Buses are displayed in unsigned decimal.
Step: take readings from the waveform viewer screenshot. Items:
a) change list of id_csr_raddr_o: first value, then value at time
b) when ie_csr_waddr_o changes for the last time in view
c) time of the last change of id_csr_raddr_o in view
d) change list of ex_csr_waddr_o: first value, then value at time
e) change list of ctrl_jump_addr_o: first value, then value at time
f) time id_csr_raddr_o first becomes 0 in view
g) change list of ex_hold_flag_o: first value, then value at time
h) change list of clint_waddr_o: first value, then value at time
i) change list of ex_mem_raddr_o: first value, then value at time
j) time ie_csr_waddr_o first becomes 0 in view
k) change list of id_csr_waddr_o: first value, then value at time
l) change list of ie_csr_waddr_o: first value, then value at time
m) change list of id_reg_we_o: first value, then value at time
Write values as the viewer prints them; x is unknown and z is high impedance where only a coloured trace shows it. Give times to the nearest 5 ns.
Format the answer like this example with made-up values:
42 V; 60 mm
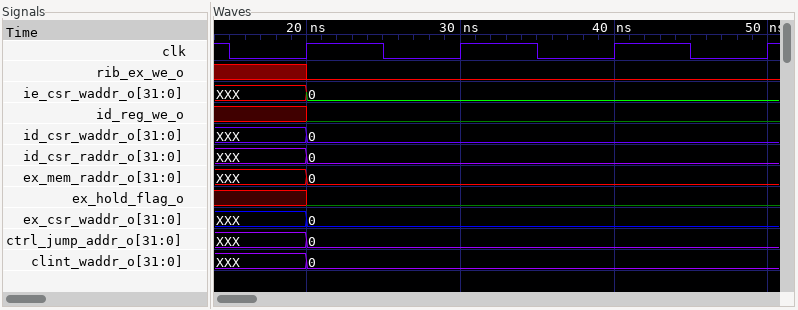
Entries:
XXX, 0 at 20 ns; 20 ns; 20 ns; XXX, 0 at 20 ns; XXX, 0 at 20 ns; 20 ns; x, 0 at 20 ns; XXX, 0 at 20 ns; XXX, 0 at 20 ns; 20 ns; XXX, 0 at 20 ns; XXX, 0 at 20 ns; x, 0 at 20 ns
